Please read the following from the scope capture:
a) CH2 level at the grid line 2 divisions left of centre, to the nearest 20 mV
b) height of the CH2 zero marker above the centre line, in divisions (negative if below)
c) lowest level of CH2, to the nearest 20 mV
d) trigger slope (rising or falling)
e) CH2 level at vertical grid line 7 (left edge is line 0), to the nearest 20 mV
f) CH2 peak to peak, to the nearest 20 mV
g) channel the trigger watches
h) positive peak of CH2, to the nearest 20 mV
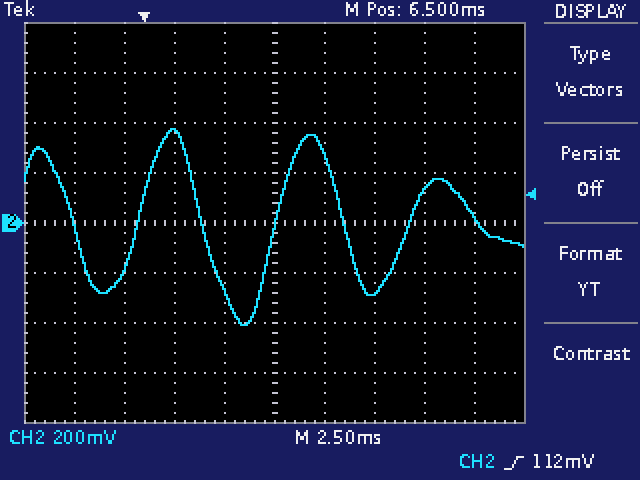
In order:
360 mV
0.0 div
-400 mV
rising
-280 mV
780 mV
CH2
380 mV
